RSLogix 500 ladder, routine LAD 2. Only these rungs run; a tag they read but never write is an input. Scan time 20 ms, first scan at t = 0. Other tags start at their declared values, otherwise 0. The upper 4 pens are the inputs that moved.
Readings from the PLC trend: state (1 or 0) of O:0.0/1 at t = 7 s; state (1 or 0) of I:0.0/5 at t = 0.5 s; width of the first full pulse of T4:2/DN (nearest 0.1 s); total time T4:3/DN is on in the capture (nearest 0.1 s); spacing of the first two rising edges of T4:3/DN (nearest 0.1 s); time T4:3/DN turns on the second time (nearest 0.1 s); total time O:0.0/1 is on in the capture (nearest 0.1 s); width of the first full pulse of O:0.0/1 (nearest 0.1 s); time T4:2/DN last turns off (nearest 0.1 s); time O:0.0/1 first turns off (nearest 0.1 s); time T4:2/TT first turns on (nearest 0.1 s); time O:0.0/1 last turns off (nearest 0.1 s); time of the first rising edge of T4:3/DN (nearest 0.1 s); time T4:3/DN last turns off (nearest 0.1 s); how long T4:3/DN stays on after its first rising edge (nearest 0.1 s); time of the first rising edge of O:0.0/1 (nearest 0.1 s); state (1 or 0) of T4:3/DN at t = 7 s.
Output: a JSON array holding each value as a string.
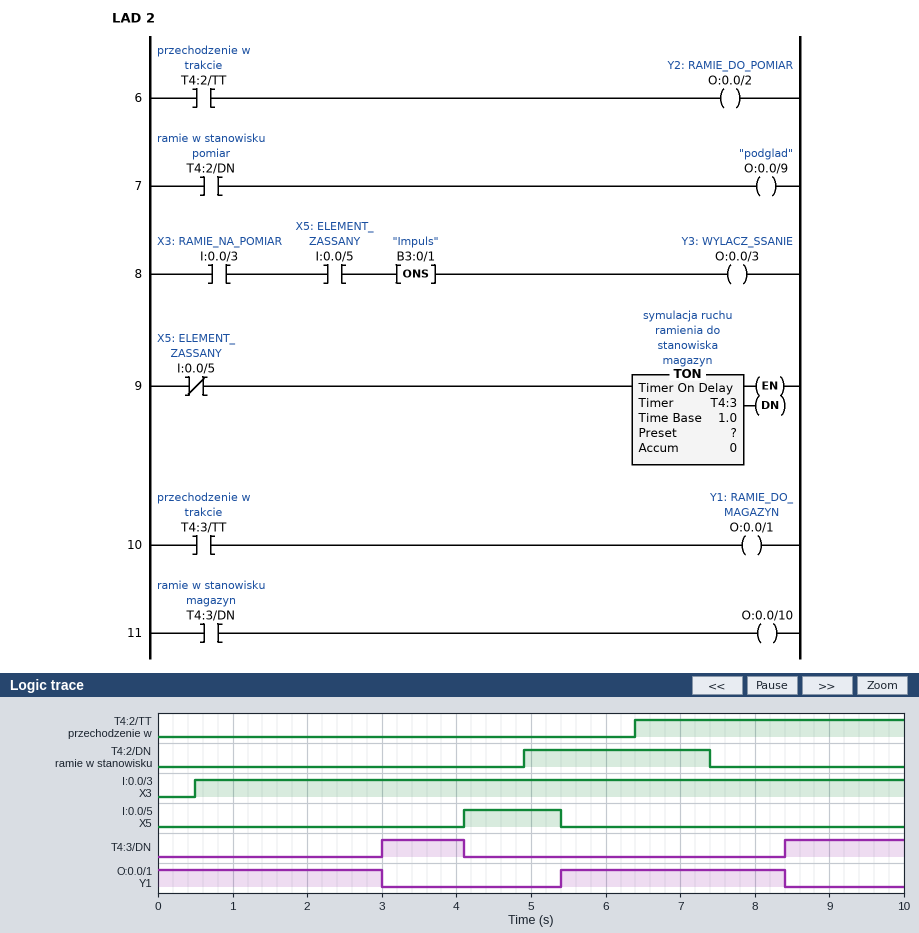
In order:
["1", "0", "2.5 s", "2.7 s", "5.4 s", "8.4 s", "6.0 s", "3.0 s", "7.4 s", "3.0 s", "6.4 s", "8.4 s", "3.0 s", "4.1 s", "1.1 s", "5.4 s", "0"]
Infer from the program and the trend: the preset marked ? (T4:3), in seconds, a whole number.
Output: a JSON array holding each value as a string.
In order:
["3 s"]
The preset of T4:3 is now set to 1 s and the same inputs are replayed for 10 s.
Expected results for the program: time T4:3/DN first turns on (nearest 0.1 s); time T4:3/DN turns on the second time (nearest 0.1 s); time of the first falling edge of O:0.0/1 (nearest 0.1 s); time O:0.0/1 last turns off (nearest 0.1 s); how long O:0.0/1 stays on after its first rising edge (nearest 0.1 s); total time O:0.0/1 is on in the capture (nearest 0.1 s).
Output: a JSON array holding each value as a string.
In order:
["1.0 s", "6.4 s", "1.0 s", "6.4 s", "1.0 s", "2.0 s"]
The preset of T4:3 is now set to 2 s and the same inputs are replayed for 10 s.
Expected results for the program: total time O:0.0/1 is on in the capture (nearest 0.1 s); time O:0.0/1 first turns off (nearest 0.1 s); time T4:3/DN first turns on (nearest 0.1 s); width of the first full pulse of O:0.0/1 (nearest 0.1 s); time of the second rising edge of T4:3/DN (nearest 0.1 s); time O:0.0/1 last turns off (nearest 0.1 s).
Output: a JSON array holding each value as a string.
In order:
["4.0 s", "2.0 s", "2.0 s", "2.0 s", "7.4 s", "7.4 s"]
